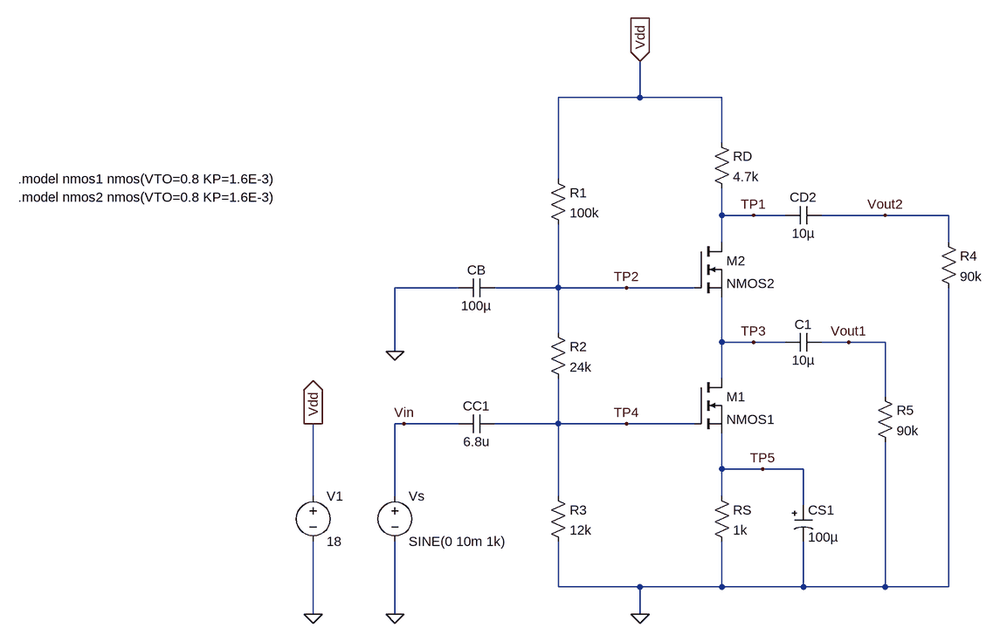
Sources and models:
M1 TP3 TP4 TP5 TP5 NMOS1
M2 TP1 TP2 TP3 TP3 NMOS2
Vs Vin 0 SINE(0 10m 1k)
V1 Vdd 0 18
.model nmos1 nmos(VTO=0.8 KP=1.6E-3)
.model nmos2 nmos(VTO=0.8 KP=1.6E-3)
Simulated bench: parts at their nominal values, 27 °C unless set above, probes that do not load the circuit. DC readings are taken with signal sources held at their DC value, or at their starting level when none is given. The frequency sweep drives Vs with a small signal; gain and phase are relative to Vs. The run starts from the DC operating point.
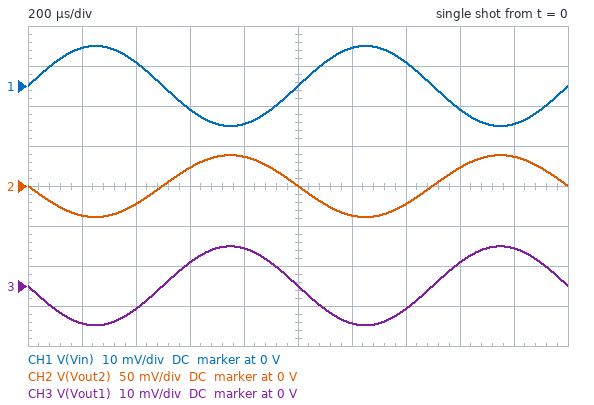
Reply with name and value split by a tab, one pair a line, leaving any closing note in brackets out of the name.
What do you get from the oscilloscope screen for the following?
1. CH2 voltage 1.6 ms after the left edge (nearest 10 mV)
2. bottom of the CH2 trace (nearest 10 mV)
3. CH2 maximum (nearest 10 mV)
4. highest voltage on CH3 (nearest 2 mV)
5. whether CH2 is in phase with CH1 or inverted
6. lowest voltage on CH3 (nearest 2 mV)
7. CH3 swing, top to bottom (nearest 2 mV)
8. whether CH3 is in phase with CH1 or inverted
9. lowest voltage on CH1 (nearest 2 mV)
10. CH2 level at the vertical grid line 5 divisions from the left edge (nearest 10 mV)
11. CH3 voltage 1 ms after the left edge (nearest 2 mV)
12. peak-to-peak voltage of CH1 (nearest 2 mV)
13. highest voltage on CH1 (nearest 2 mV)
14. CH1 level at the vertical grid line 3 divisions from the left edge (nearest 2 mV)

CH2 voltage 1.6 ms after the left edge	20 mV
bottom of the CH2 trace	-40 mV
CH2 maximum	40 mV
highest voltage on CH3	10 mV
whether CH2 is in phase with CH1 or inverted	inverted
lowest voltage on CH3	-10 mV
CH3 swing, top to bottom	20 mV
whether CH3 is in phase with CH1 or inverted	inverted
lowest voltage on CH1	-10 mV
CH2 level at the vertical grid line 5 divisions from the left edge	0 V
CH3 voltage 1 ms after the left edge	0 V
peak-to-peak voltage of CH1	20 mV
highest voltage on CH1	10 mV
CH1 level at the vertical grid line 3 divisions from the left edge	-6 mV
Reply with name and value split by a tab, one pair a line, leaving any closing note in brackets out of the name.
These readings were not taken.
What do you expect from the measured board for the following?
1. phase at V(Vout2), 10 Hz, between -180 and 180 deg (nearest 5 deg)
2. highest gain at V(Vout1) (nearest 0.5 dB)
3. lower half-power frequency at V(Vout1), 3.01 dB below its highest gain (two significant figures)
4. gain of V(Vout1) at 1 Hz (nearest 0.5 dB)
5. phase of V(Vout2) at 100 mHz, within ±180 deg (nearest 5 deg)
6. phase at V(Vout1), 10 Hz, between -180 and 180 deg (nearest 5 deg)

phase at V(Vout2), 10 Hz, between -180 and 180 deg	-155 deg
highest gain at V(Vout1)	0 dB
lower half-power frequency at V(Vout1), 3.01 dB below its highest gain	4.1 Hz
gain of V(Vout1) at 1 Hz	-14.5 dB
phase of V(Vout2) at 100 mHz, within ±180 deg	-40 deg
phase at V(Vout1), 10 Hz, between -180 and 180 deg	-155 deg
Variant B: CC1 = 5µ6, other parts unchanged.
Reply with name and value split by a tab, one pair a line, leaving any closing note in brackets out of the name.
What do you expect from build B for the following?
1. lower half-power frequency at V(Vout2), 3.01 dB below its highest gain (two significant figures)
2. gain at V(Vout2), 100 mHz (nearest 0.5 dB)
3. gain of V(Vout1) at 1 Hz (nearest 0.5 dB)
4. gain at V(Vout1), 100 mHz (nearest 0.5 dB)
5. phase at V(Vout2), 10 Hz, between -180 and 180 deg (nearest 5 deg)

lower half-power frequency at V(Vout2), 3.01 dB below its highest gain	4.7 Hz
gain at V(Vout2), 100 mHz	-29.5 dB
gain of V(Vout1) at 1 Hz	-16.0 dB
gain at V(Vout1), 100 mHz	-43.0 dB
phase at V(Vout2), 10 Hz, between -180 and 180 deg	-150 deg
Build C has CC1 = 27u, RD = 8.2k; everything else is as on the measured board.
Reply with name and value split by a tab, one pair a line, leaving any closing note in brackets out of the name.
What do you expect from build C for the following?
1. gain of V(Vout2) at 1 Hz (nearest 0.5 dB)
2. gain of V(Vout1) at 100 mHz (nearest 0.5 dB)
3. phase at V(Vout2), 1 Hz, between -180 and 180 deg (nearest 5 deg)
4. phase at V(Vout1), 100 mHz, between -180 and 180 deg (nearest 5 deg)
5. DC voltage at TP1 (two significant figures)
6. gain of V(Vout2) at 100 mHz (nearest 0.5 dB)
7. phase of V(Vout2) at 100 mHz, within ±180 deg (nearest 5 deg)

gain of V(Vout2) at 1 Hz	9.5 dB
gain of V(Vout1) at 100 mHz	-29.5 dB
phase at V(Vout2), 1 Hz, between -180 and 180 deg	-120 deg
phase at V(Vout1), 100 mHz, between -180 and 180 deg	15 deg
DC voltage at TP1	16 V
gain of V(Vout2) at 100 mHz	-11.5 dB
phase of V(Vout2) at 100 mHz, within ±180 deg	-45 deg
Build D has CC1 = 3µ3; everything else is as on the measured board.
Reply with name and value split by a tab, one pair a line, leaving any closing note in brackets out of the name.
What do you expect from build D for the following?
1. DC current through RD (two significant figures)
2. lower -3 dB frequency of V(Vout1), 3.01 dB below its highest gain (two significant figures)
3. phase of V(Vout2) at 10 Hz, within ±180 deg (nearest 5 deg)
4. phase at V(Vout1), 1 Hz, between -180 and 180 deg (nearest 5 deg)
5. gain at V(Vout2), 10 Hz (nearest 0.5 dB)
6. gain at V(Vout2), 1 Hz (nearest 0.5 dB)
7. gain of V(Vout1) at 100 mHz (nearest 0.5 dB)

DC current through RD	240 µA
lower -3 dB frequency of V(Vout1), 3.01 dB below its highest gain	6.9 Hz
phase of V(Vout2) at 10 Hz, within ±180 deg	-140 deg
phase at V(Vout1), 1 Hz, between -180 and 180 deg	-70 deg
gain at V(Vout2), 10 Hz	10.0 dB
gain at V(Vout2), 1 Hz	-8.5 dB
gain of V(Vout1) at 100 mHz	-47.5 dB
